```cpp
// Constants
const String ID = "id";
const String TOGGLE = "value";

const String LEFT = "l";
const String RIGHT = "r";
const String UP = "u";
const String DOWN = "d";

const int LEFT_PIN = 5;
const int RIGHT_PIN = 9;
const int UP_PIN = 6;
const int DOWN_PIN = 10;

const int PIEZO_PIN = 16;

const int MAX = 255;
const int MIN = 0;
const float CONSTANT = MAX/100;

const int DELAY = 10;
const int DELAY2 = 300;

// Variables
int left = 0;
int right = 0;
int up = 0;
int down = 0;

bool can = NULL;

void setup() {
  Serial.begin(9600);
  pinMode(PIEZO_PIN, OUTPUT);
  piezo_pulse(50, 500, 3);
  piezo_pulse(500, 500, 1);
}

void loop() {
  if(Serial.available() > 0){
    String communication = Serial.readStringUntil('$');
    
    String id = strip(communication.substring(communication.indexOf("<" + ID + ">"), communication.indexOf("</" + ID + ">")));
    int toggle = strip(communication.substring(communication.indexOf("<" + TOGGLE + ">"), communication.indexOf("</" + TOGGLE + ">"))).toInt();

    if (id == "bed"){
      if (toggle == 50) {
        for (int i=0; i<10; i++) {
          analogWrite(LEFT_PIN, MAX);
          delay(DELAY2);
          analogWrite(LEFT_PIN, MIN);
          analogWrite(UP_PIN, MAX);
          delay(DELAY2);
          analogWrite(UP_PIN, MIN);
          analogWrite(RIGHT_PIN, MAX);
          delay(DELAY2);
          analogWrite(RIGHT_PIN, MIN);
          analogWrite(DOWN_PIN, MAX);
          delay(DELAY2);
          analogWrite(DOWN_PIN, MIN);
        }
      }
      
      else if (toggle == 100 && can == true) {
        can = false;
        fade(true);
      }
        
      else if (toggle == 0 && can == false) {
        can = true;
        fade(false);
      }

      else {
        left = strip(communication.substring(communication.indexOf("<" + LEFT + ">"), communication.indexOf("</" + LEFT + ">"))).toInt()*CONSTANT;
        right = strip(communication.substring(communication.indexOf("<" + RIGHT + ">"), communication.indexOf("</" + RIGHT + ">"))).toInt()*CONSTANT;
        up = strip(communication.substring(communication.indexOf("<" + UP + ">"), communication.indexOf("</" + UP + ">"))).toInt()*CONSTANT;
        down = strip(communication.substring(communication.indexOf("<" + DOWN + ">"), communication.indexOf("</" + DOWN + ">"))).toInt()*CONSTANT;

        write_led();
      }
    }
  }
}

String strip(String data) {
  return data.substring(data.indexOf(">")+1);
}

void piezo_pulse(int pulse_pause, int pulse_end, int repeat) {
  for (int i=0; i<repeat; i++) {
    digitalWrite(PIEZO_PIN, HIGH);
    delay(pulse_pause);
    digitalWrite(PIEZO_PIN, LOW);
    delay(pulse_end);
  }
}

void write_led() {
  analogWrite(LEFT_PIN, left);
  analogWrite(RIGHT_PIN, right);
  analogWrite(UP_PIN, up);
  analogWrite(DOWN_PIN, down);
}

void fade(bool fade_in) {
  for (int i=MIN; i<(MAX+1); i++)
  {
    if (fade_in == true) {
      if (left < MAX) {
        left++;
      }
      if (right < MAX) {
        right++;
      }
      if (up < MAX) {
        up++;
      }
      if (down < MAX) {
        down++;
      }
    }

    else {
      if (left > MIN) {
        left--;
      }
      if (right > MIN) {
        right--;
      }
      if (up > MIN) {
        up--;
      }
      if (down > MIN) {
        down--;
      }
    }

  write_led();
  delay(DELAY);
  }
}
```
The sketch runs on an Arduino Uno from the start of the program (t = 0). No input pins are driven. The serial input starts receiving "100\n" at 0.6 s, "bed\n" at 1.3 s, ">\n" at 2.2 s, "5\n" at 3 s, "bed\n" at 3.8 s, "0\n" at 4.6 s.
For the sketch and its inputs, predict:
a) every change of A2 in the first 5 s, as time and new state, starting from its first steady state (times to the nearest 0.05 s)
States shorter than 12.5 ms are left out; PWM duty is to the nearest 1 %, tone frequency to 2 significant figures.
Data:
0 s high; 0.05 s low; 0.55 s high; 0.6 s low; 1.1 s high; 1.15 s low; 1.65 s high; 2.15 s low
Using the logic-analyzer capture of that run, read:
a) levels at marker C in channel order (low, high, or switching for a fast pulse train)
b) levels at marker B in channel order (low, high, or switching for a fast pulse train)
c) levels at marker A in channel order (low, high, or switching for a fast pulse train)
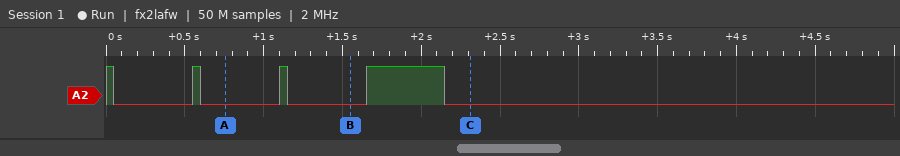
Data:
A2 low
A2 low
A2 low
